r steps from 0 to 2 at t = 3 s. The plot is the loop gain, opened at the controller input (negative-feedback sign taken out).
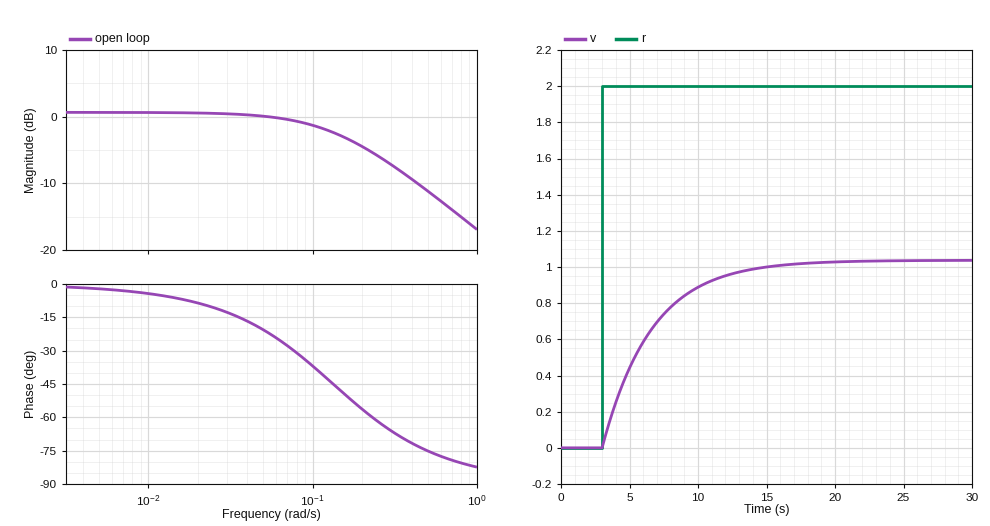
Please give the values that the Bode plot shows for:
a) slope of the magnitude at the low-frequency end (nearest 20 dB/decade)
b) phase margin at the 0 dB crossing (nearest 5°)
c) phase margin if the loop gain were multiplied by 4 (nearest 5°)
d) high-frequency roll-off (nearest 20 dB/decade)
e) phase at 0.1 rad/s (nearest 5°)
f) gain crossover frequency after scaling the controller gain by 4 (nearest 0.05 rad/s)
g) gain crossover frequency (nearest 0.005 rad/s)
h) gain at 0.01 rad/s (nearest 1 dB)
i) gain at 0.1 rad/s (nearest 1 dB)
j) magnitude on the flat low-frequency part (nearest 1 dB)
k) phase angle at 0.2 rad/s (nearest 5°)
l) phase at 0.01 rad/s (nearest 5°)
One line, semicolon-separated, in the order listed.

0 dB/decade; 160°; 105°; -20 dB/decade; -35°; 0.55 rad/s; 0.055 rad/s; 1 dB; -1 dB; 1 dB; -55°; -5°
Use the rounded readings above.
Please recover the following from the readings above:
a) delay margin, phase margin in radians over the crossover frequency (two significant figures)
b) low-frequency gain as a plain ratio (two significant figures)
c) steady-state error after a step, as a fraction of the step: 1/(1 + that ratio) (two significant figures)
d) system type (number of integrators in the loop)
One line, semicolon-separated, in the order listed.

51 s; 1.1; 0.48; 0
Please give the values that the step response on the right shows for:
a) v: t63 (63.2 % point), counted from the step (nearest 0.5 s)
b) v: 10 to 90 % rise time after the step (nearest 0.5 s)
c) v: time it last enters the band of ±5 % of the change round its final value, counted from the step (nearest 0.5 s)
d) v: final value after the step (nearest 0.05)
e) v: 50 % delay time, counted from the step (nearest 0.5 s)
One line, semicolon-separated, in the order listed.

3.5 s; 8.0 s; 11.0 s; 1.05; 2.5 s
